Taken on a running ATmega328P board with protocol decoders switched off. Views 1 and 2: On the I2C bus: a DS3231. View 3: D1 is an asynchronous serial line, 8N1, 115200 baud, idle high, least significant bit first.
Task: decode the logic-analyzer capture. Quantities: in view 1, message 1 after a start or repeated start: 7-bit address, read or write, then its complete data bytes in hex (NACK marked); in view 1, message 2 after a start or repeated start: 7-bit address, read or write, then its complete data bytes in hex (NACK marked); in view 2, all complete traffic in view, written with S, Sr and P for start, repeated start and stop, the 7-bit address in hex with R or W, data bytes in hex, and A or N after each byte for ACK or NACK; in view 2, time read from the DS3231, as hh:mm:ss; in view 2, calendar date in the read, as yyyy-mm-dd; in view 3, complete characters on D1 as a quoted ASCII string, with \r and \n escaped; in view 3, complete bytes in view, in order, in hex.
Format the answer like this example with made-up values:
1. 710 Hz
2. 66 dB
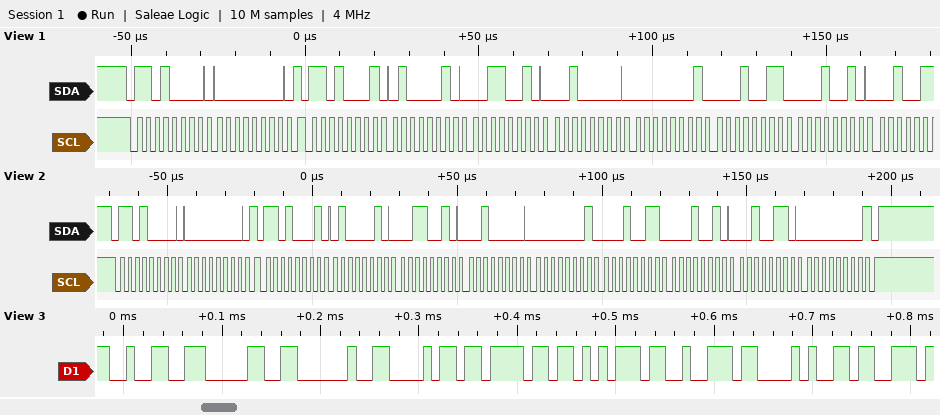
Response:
1. 0x68 write: 00
2. 0x68 read: 42 32 20 01 13 12
3. S 68W A 00 A Sr 68R A 42 A 32 A 20 A 01 A 13 A 12 A 26 A 00 N P
4. 20:32:42
5. 2026-12-13
6. "20 hour(s"
7. 32 30 20 68 6F 75 72 28 73
